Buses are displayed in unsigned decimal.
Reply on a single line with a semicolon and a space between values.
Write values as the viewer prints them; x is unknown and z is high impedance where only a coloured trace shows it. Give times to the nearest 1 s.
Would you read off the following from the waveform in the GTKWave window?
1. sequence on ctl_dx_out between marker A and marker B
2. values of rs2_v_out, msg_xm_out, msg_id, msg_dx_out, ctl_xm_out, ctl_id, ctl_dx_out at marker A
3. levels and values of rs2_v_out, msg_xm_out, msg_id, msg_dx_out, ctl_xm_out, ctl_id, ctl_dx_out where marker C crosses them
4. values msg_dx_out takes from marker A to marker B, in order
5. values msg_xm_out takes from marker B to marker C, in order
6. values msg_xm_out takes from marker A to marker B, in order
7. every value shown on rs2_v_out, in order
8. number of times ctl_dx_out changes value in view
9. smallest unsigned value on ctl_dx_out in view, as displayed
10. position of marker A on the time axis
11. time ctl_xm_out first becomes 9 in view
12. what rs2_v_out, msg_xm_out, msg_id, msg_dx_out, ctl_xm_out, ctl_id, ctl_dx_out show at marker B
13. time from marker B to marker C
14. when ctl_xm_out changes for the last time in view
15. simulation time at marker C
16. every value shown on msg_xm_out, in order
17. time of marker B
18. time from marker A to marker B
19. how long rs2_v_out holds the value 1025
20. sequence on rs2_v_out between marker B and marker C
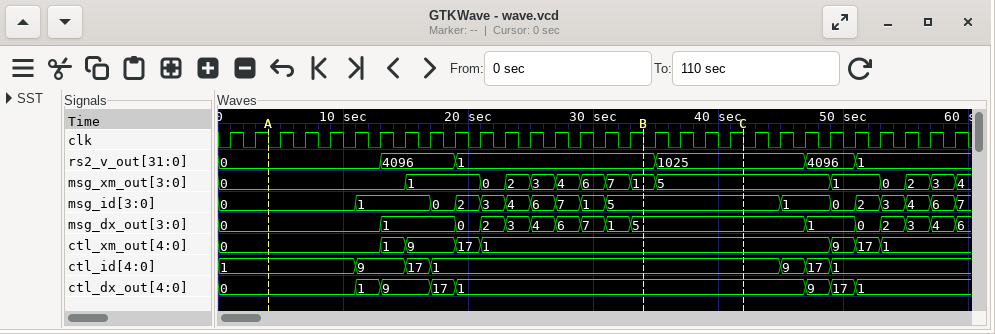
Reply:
0, 1, 9, 17, 1; rs2_v_out=0, msg_xm_out=0, msg_id=0, msg_dx_out=0, ctl_xm_out=0, ctl_id=1, ctl_dx_out=0; rs2_v_out=1025, msg_xm_out=5, msg_id=5, msg_dx_out=5, ctl_xm_out=1, ctl_id=1, ctl_dx_out=1; 0, 1, 0, 2, 3, 4, 6, 7, 1, 5; 1, 5; 0, 1, 0, 2, 3, 4, 6, 7, 1; 0, 4096, 1, 1025, 4096, 1; 7; 0; 4 s; 15 s; rs2_v_out=1, msg_xm_out=1, msg_id=5, msg_dx_out=5, ctl_xm_out=1, ctl_id=1, ctl_dx_out=1; 8 s; 53 s; 42 s; 0, 1, 0, 2, 3, 4, 6, 7, 1, 5, 1, 0, 2, 3, 4; 34 s; 30 s; 12 s; 1, 1025
